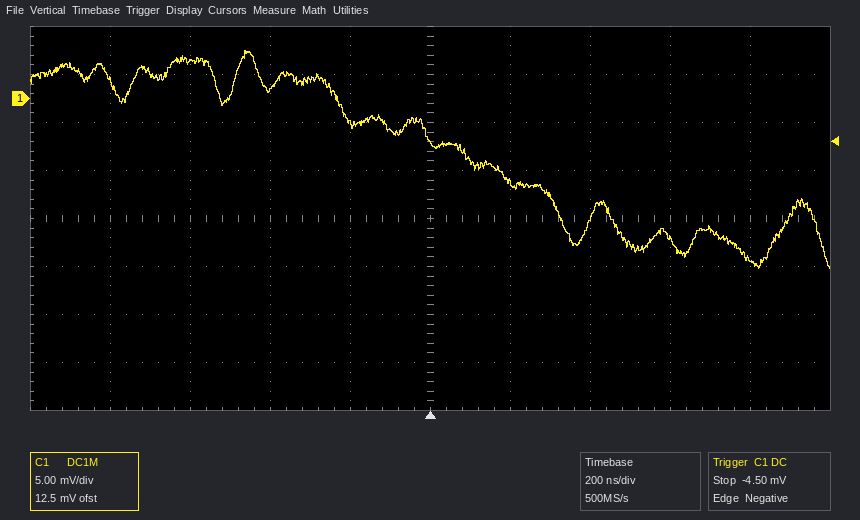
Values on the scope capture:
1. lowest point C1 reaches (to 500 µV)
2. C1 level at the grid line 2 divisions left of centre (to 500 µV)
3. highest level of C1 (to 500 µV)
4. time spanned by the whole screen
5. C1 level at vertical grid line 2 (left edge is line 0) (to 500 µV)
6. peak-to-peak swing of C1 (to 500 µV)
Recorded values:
-17.5 mV
1.0 mV
5.0 mV
2 µs
4.0 mV
22.5 mV
